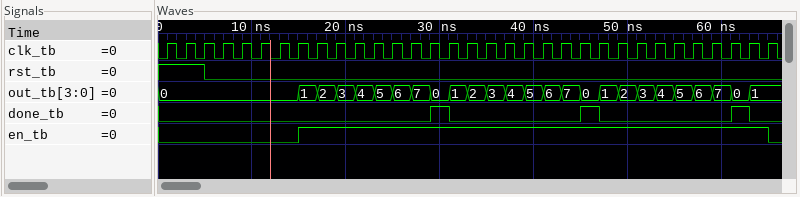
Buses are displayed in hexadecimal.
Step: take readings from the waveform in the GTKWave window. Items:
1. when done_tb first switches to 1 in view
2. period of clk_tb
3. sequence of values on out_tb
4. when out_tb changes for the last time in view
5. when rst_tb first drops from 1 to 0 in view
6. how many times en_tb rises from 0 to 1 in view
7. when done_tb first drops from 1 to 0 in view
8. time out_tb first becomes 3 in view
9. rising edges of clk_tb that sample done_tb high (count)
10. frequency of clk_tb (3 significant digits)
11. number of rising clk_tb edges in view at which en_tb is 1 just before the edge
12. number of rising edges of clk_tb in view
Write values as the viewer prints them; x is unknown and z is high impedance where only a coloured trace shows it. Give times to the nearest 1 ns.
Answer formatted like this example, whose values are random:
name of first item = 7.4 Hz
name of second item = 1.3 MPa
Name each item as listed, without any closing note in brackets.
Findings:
when done_tb first switches to 1 in view = 29 ns
period of clk_tb = 2 ns
sequence of values on out_tb = 0, 1, 2, 3, 4, 5, 6, 7, 0, 1, 2, 3, 4, 5, 6, 7, 0, 1, 2, 3, 4, 5, 6, 7, 0, 1
when out_tb changes for the last time in view = 63 ns
when rst_tb first drops from 1 to 0 in view = 5 ns
how many times en_tb rises from 0 to 1 in view = 1
when done_tb first drops from 1 to 0 in view = 31 ns
time out_tb first becomes 3 in view = 19 ns
rising edges of clk_tb that sample done_tb high = 3
frequency of clk_tb = 500 MHz
number of rising clk_tb edges in view at which en_tb is 1 just before the edge = 25
number of rising edges of clk_tb in view = 33
